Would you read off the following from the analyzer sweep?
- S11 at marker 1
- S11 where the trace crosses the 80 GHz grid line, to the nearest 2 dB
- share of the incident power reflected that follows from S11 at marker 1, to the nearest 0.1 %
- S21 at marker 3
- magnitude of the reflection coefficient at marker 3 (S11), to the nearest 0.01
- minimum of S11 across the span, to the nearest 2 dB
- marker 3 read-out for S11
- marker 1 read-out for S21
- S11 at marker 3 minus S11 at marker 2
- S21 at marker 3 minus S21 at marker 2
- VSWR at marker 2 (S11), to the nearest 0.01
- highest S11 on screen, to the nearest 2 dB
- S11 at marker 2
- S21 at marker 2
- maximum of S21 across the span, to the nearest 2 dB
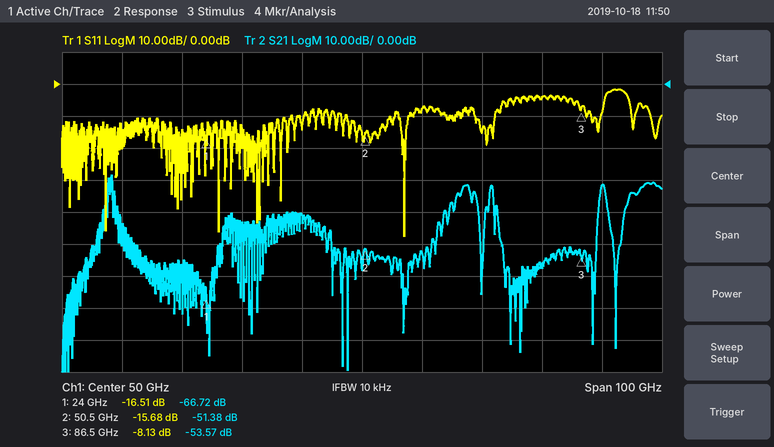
-16.51 dB
-4 dB
2.2 %
-53.57 dB
0.39
-48 dB
-8.13 dB
-66.72 dB
7.55 dB
-2.19 dB
1.39
-2 dB
-15.68 dB
-51.38 dB
-28 dB
